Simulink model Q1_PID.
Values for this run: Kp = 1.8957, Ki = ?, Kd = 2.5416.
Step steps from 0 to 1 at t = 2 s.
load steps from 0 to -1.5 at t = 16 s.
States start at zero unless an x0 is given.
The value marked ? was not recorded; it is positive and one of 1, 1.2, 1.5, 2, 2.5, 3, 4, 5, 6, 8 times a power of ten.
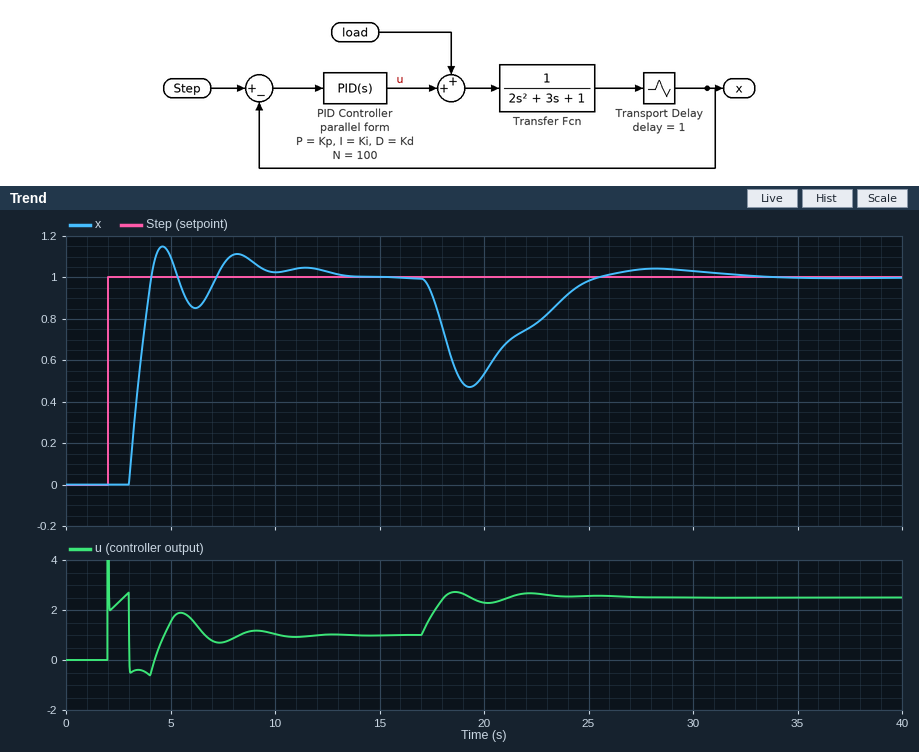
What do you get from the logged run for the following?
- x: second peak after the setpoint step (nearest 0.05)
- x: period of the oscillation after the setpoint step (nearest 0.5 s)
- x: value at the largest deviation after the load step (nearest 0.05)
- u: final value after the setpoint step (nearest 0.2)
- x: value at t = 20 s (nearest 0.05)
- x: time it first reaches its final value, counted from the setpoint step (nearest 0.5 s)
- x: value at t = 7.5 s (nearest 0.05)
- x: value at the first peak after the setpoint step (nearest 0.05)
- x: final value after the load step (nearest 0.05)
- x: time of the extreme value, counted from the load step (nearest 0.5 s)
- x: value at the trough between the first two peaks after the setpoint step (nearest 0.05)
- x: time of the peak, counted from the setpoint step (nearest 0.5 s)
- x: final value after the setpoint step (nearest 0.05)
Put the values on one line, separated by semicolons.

1.10; 3.5 s; 0.45; 1.0; 0.55; 2.0 s; 1.05; 1.15; 1.00; 3.5 s; 0.85; 2.5 s; 1.00
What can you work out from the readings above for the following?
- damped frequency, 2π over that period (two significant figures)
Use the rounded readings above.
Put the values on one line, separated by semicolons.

1.8 rad/s
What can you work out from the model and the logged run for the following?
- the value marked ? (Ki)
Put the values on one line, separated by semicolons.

0.8
